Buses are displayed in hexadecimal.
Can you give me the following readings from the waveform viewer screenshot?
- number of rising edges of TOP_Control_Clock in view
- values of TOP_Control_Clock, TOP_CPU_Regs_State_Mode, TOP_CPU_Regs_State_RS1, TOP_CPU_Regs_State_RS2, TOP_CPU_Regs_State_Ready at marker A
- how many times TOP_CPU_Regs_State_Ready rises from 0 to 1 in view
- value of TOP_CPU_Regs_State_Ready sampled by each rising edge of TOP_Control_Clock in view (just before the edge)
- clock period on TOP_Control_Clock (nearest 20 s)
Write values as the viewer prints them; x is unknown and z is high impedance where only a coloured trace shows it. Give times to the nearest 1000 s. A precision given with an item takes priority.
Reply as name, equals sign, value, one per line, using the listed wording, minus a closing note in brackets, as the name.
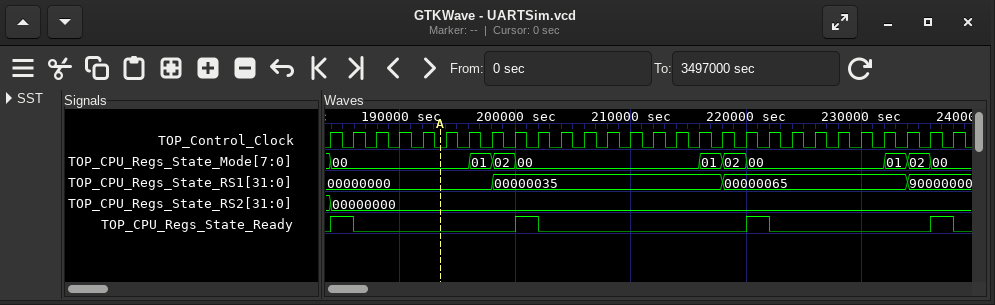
number of rising edges of TOP_Control_Clock in view = 28
values of TOP_Control_Clock, TOP_CPU_Regs_State_Mode, TOP_CPU_Regs_State_RS1, TOP_CPU_Regs_State_RS2, TOP_CPU_Regs_State_Ready at marker A = TOP_Control_Clock=0, TOP_CPU_Regs_State_Mode=00, TOP_CPU_Regs_State_RS1=00000000, TOP_CPU_Regs_State_RS2=00000000, TOP_CPU_Regs_State_Ready=0
how many times TOP_CPU_Regs_State_Ready rises from 0 to 1 in view = 4
value of TOP_CPU_Regs_State_Ready sampled by each rising edge of TOP_Control_Clock in view = 0 1 0 0 0 0 0 0 0 1 0 0 0 0 0 0 0 0 0 1 0 0 0 0 0 0 0 1
clock period on TOP_Control_Clock = 2000 s
